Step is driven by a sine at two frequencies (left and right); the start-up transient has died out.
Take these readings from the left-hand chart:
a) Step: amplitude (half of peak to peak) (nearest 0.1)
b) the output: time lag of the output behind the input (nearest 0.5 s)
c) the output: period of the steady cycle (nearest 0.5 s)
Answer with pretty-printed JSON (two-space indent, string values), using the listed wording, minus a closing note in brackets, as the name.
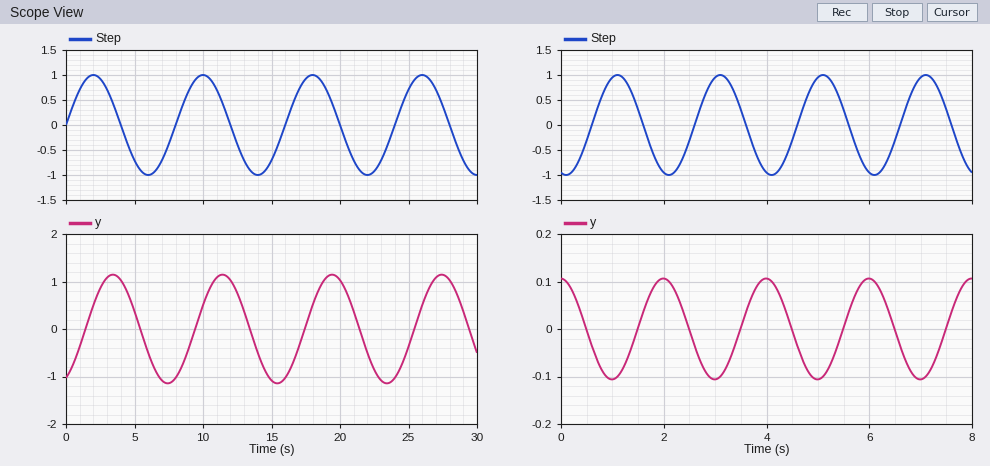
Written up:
{
  "Step: amplitude (half of peak to peak)": "1.0",
  "the output: time lag of the output behind the input": "1.5 s",
  "the output: period of the steady cycle": "8.0 s"
}
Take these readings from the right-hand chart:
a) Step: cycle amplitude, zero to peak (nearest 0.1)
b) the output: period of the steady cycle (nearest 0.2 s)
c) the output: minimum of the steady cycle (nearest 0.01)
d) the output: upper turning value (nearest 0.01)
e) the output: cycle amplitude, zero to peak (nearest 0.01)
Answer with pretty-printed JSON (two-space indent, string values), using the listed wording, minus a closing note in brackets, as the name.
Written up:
{
  "Step: cycle amplitude, zero to peak": "1.0",
  "the output: period of the steady cycle": "2.0 s",
  "the output: minimum of the steady cycle": "-0.11",
  "the output: upper turning value": "0.11",
  "the output: cycle amplitude, zero to peak": "0.11"
}
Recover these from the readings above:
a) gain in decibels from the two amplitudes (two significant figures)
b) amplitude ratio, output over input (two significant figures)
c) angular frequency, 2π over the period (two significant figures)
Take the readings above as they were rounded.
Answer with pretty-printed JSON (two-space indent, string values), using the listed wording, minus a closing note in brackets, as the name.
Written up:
{
  "gain in decibels from the two amplitudes": "-19 dB",
  "amplitude ratio, output over input": "0.11",
  "angular frequency, 2π over the period": "3.1 rad/s"
}
